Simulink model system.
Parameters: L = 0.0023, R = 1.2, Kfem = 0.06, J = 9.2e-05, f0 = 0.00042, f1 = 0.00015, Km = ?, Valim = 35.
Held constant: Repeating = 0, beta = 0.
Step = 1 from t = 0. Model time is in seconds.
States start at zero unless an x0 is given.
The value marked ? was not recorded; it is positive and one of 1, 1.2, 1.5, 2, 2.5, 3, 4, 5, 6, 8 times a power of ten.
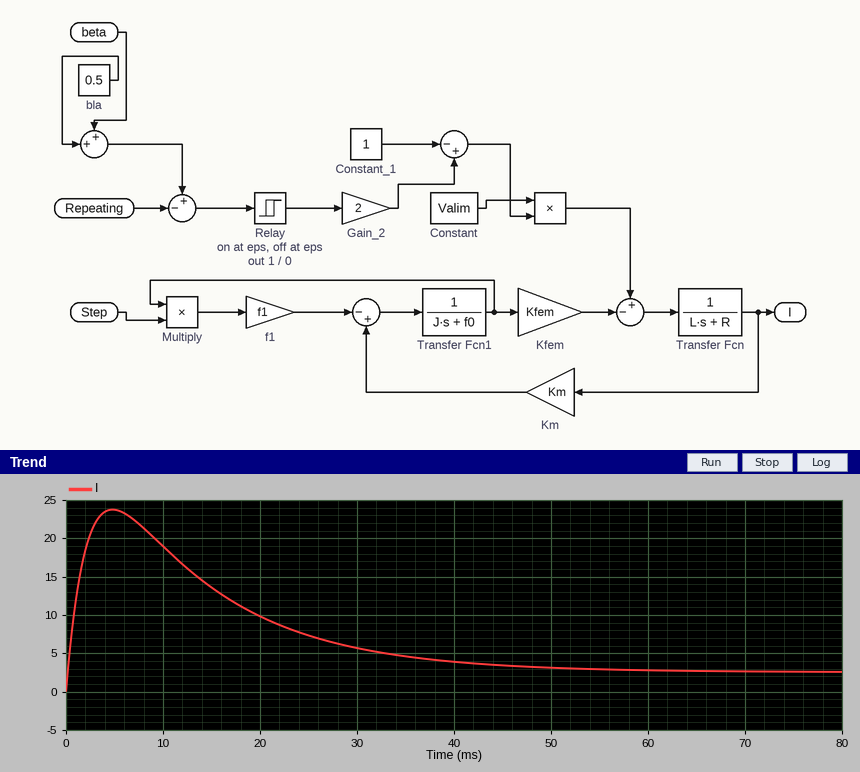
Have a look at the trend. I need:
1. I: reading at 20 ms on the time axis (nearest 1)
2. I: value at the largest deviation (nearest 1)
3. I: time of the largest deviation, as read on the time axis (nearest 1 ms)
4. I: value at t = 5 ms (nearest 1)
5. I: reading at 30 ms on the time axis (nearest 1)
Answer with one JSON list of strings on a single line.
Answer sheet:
["10", "24", "5 ms", "24", "6"]
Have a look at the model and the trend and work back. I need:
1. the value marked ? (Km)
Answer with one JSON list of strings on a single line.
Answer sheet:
["0.12"]
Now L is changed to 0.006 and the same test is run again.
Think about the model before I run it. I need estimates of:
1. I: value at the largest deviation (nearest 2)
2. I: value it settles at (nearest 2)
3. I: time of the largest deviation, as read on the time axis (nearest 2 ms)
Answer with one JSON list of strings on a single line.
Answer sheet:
["20", "2", "10 ms"]
